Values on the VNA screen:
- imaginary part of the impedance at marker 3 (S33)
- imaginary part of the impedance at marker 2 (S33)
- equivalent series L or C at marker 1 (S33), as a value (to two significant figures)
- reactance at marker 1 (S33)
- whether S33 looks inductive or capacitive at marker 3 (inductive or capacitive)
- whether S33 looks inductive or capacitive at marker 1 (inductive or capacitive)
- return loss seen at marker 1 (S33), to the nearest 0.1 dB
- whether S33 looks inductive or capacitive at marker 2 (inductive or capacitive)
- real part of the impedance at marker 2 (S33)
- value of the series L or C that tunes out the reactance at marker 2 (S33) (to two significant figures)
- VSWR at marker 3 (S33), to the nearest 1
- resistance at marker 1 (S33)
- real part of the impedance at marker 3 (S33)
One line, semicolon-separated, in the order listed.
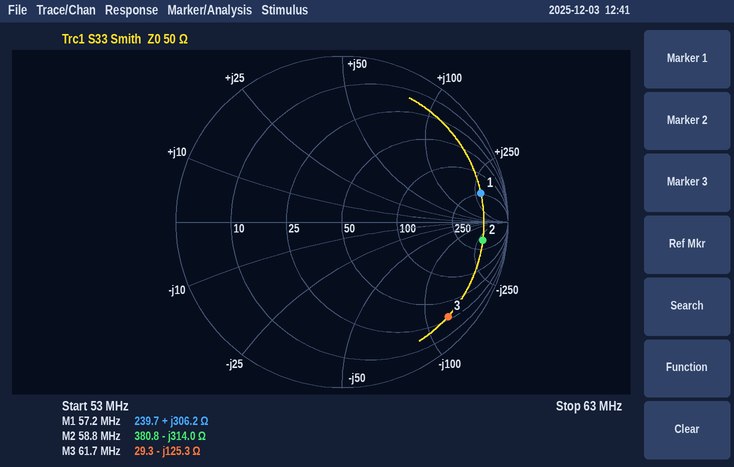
-125.3 Ω; -314.0 Ω; 850 nH; +306.2 Ω; capacitive; inductive; 1.4 dB; capacitive; 380.8 Ω; 850 nH; 13; 239.7 Ω; 29.3 Ω
